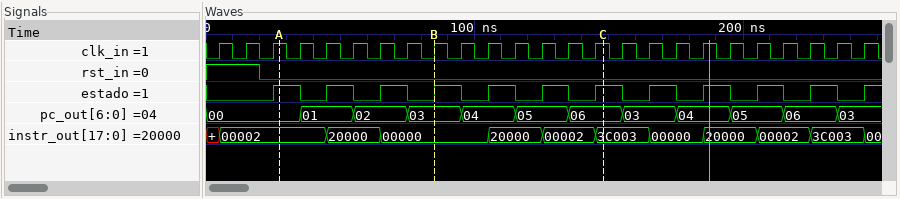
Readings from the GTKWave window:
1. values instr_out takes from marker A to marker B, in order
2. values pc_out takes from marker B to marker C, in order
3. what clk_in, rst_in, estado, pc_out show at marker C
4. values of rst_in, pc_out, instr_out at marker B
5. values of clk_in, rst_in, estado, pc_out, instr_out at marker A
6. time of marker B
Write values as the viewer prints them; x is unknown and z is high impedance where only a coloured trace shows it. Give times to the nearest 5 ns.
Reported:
00002, 20000, 00000
03, 04, 05, 06
clk_in=1, rst_in=0, estado=1, pc_out=06
rst_in=0, pc_out=03, instr_out=00000
clk_in=1, rst_in=0, estado=1, pc_out=00, instr_out=00002
85 ns
